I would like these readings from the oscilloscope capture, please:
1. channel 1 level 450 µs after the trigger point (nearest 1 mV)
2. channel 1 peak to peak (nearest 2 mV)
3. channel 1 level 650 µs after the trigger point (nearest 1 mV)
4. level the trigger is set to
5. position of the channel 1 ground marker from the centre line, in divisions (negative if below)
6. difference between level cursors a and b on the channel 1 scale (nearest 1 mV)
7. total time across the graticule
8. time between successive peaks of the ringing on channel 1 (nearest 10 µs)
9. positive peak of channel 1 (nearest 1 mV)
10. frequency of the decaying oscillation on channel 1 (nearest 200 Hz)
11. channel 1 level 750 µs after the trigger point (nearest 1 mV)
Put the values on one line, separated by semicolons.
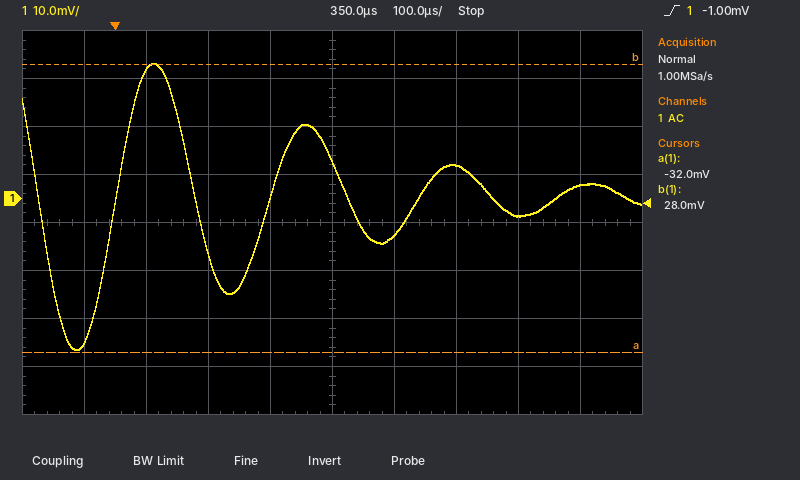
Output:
-8 mV; 60 mV; -4 mV; -1.00 mV; +0.5 div; 60 mV; 1 ms; 240 µs; 28 mV; 4.2 kHz; 3 mV
